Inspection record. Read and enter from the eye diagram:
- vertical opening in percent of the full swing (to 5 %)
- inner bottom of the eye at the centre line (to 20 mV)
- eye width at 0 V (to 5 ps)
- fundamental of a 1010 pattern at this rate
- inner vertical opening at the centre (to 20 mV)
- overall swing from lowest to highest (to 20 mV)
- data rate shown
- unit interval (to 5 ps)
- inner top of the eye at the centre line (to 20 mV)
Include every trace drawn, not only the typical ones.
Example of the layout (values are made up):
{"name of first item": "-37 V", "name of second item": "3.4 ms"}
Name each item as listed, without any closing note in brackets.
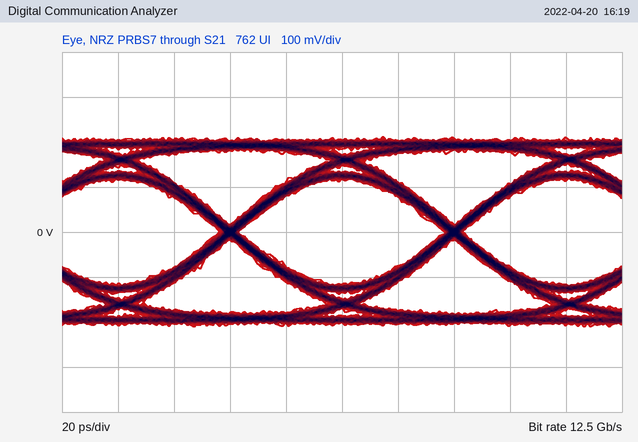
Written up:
{"vertical opening in percent of the full swing": "55 %", "inner bottom of the eye at the centre line": "-120 mV", "eye width at 0 V": "75 ps", "fundamental of a 1010 pattern at this rate": "6.25 GHz", "inner vertical opening at the centre": "240 mV", "overall swing from lowest to highest": "420 mV", "data rate shown": "12.5 Gb/s", "unit interval": "80 ps", "inner top of the eye at the centre line": "120 mV"}
